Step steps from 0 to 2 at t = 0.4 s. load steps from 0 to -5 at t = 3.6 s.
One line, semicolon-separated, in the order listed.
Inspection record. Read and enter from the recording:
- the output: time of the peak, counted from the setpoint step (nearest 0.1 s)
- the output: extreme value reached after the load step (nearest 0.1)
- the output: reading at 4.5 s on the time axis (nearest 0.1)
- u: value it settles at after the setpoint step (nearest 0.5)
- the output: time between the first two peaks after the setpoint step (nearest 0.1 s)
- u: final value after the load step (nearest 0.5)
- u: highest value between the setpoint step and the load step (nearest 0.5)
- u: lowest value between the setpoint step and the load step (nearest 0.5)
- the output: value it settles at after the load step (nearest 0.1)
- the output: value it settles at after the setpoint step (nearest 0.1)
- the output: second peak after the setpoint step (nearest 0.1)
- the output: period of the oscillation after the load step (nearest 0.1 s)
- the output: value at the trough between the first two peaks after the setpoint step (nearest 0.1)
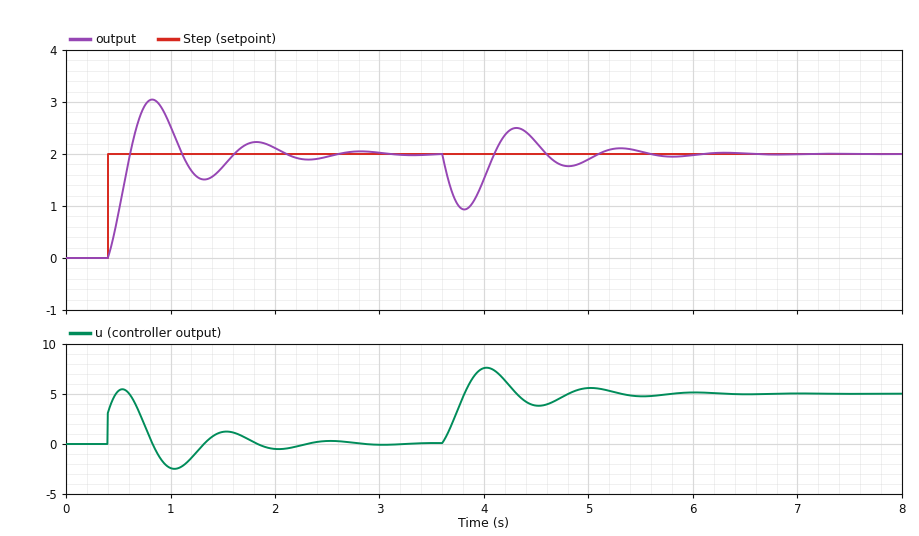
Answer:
0.4 s; 0.9; 2.2; 0.0; 1.0 s; 5.0; 5.5; -2.5; 2.0; 2.0; 2.2; 1.0 s; 1.5
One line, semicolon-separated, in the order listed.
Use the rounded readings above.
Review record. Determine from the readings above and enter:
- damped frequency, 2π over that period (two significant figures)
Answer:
6.3 rad/s
